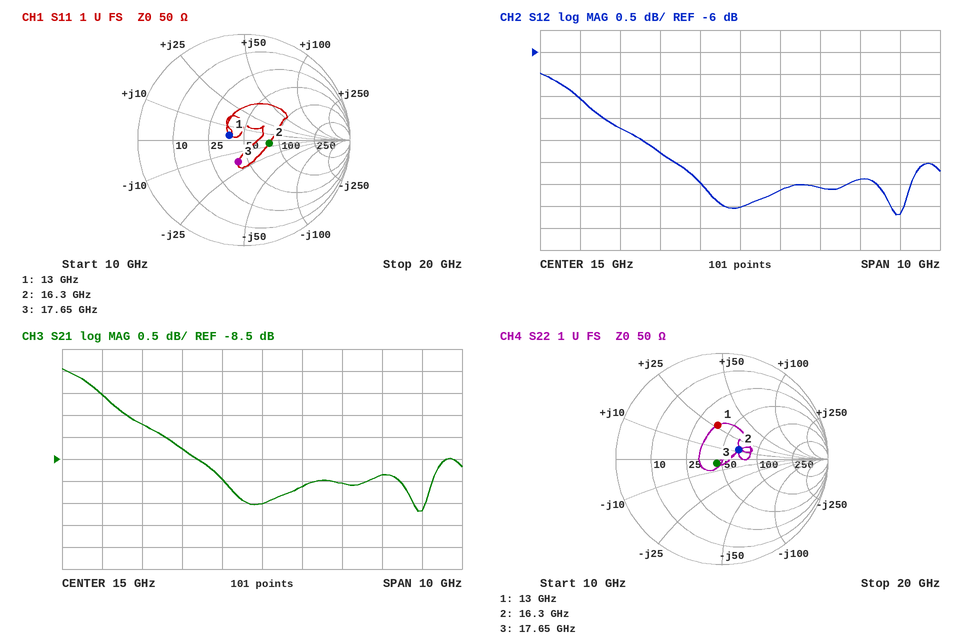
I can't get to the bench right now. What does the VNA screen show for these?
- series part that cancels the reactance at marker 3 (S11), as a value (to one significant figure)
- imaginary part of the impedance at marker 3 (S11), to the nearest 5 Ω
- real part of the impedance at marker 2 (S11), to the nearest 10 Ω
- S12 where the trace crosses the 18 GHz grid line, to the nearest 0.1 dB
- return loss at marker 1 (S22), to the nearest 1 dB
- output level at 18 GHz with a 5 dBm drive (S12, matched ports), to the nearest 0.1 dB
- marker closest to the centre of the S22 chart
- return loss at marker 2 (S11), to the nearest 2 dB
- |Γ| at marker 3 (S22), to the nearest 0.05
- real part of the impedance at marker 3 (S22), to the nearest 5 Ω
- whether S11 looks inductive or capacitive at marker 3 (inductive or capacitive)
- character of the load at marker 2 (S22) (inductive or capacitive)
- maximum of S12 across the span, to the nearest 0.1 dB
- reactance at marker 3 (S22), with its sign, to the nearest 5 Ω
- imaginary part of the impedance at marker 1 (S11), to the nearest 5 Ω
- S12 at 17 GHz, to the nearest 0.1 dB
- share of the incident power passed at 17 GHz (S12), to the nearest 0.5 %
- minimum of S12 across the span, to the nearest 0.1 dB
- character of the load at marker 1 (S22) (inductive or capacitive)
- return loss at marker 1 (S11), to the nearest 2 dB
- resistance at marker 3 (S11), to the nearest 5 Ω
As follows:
200 pH
-20 Ω
80 Ω
-8.9 dB
10 dB
-3.9 dBm
marker 3
12 dB
0.05
45 Ω
capacitive
inductive
-6.5 dB
-5 Ω
+5 Ω
-9.1 dB
12.5 %
-9.7 dB
inductive
16 dB
40 Ω
